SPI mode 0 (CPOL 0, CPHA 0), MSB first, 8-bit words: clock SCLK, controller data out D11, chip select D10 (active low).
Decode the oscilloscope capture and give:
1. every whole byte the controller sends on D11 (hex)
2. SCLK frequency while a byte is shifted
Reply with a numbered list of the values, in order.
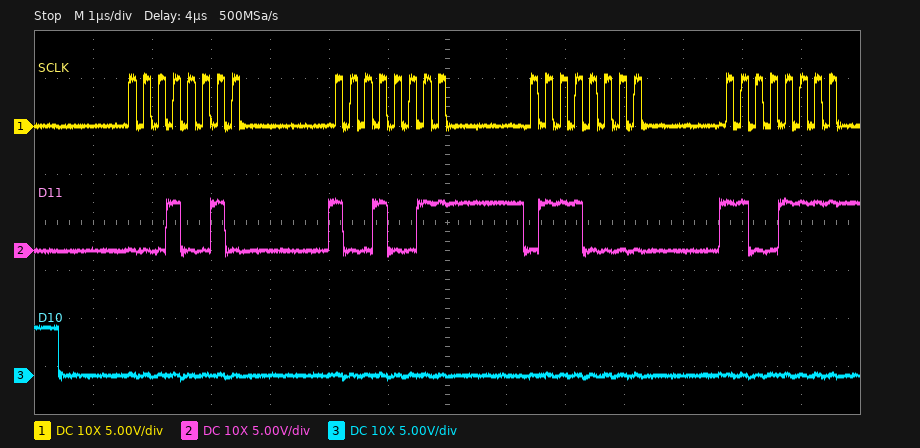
1. 0x12 0x93 0x70 0xCF
2. 4 MHz
